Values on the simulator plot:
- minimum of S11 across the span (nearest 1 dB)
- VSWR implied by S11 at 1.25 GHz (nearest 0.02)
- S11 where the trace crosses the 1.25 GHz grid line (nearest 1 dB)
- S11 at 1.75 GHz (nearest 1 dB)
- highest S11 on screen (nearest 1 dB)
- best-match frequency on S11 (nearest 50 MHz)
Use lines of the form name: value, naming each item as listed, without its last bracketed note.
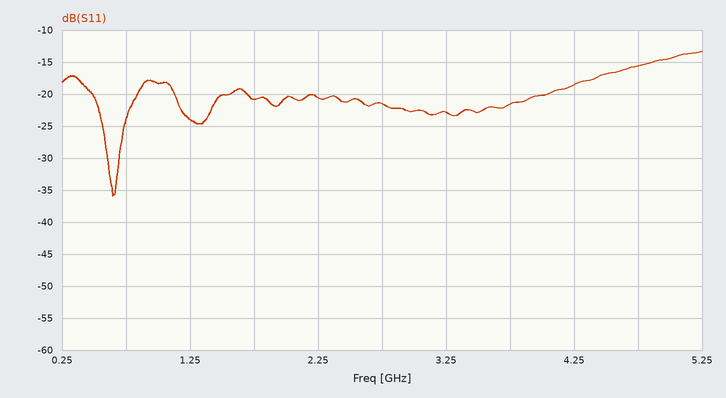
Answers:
minimum of S11 across the span: -36 dB
VSWR implied by S11 at 1.25 GHz: 1.14
S11 where the trace crosses the 1.25 GHz grid line: -24 dB
S11 at 1.75 GHz: -21 dB
highest S11 on screen: -13 dB
best-match frequency on S11: 650 MHz
